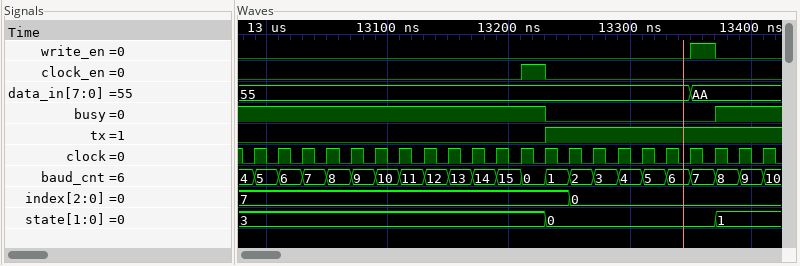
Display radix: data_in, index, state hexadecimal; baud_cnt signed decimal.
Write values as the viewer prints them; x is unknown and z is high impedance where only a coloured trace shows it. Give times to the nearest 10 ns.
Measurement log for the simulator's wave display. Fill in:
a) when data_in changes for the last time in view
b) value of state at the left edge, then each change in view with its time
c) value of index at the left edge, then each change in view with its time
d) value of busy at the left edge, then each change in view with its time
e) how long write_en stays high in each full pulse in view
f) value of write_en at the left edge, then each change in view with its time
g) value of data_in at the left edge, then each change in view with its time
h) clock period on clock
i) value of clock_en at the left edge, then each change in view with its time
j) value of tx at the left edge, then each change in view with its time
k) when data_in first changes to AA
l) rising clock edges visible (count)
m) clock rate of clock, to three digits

13350 ns
3, 0 at 13230 ns, 1 at 13370 ns
7, 0 at 13250 ns
1, 0 at 13230 ns, 1 at 13370 ns
20 ns
0, 1 at 13350 ns, 0 at 13370 ns
55, AA at 13350 ns
20 ns
0, 1 at 13210 ns, 0 at 13230 ns
0, 1 at 13230 ns
13350 ns
22
50.0 MHz
